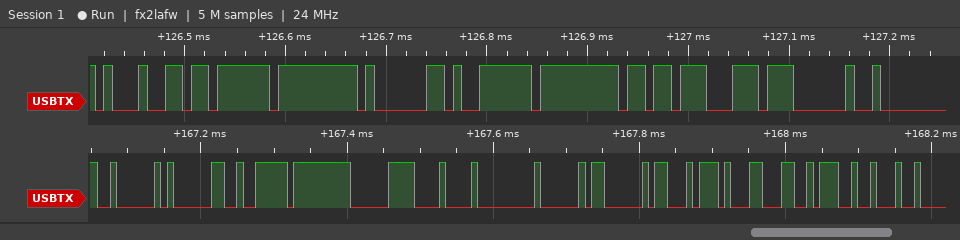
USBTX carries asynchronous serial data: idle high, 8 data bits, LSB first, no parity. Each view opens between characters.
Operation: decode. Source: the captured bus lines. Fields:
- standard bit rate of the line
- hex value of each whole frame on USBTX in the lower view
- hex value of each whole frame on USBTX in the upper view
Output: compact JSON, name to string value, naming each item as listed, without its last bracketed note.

{"standard bit rate of the line": "115200 baud", "hex value of each whole frame on USBTX in the lower view": "02, 81, F2, FF, E0, 08, 00, A0, A0, 74, 8C, 3A, 22", "hex value of each whole frame on USBTX in the upper view": "91, FB, FF, 81, F9, FF, DB, DC, 20"}
